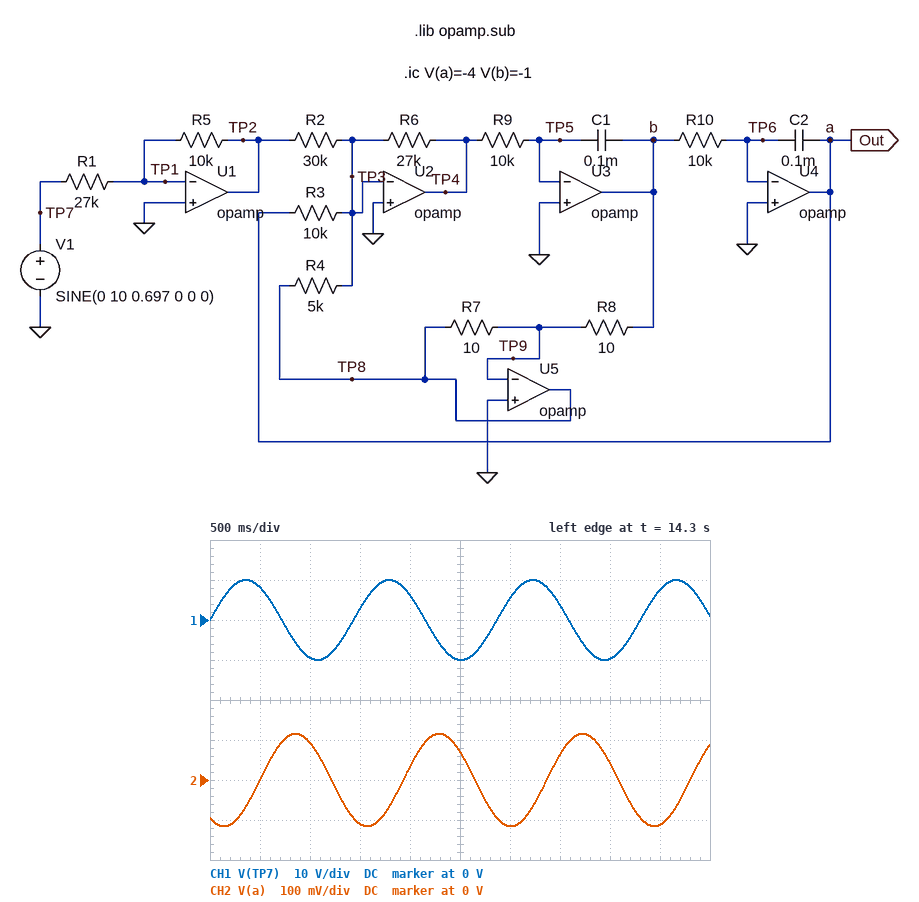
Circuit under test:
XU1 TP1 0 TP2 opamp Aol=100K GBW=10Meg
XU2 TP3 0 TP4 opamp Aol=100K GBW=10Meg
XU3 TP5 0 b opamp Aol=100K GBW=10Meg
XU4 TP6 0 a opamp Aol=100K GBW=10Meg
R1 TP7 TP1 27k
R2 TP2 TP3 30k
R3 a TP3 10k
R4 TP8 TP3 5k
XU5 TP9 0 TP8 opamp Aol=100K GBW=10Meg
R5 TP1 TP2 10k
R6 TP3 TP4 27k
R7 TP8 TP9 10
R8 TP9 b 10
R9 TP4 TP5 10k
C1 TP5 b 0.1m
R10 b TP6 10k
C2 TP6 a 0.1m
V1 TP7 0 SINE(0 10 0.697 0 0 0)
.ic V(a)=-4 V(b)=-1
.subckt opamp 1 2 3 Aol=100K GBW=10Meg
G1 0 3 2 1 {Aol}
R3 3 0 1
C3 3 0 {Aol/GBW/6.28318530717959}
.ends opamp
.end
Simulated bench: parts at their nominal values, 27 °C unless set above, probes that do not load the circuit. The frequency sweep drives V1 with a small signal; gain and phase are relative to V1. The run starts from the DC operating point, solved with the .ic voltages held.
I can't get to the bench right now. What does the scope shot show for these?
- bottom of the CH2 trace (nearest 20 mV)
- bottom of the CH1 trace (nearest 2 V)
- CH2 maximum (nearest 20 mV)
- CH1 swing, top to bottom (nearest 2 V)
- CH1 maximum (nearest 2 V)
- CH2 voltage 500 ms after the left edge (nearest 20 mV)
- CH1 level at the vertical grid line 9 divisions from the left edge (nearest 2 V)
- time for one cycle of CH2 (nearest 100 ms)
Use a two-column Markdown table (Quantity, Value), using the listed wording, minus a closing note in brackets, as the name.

| Quantity | Value |
|---|---|
| bottom of the CH2 trace | -120 mV |
| bottom of the CH1 trace | -10 V |
| CH2 maximum | 120 mV |
| CH1 swing, top to bottom | 20 V |
| CH1 maximum | 10 V |
| CH2 voltage 500 ms after the left edge | 0 V |
| CH1 level at the vertical grid line 9 divisions from the left edge | 8 V |
| time for one cycle of CH2 | 1.4 s |
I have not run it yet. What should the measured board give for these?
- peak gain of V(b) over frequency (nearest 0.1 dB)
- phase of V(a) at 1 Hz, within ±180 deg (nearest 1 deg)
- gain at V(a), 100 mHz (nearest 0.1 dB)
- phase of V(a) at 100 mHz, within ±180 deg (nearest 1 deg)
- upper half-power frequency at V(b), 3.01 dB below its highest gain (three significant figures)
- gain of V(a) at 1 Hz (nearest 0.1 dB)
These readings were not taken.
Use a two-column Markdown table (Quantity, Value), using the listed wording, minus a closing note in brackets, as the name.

| Quantity | Value |
|---|---|
| peak gain of V(b) over frequency | -24.2 dB |
| phase of V(a) at 1 Hz, within ±180 deg | -137 deg |
| gain at V(a), 100 mHz | -21.8 dB |
| phase of V(a) at 100 mHz, within ±180 deg | -56 deg |
| upper half-power frequency at V(b), 3.01 dB below its highest gain | 933 mHz |
| gain of V(a) at 1 Hz | -43.5 dB |
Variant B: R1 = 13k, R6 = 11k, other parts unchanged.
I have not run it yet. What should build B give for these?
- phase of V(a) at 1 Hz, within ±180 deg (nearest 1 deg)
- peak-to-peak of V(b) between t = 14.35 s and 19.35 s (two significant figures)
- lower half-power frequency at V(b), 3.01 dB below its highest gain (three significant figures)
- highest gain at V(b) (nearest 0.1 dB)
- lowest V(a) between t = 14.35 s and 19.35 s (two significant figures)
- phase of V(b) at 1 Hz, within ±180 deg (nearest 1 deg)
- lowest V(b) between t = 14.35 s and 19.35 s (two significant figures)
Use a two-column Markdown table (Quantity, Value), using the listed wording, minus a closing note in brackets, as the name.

| Quantity | Value |
|---|---|
| phase of V(a) at 1 Hz, within ±180 deg | -160 deg |
| peak-to-peak of V(b) between t = 14.35 s and 19.35 s | 1.2 V |
| lower half-power frequency at V(b), 3.01 dB below its highest gain | 66.8 mHz |
| highest gain at V(b) | -17.8 dB |
| lowest V(a) between t = 14.35 s and 19.35 s | -140 mV |
| phase of V(b) at 1 Hz, within ±180 deg | 110 deg |
| lowest V(b) between t = 14.35 s and 19.35 s | -600 mV |
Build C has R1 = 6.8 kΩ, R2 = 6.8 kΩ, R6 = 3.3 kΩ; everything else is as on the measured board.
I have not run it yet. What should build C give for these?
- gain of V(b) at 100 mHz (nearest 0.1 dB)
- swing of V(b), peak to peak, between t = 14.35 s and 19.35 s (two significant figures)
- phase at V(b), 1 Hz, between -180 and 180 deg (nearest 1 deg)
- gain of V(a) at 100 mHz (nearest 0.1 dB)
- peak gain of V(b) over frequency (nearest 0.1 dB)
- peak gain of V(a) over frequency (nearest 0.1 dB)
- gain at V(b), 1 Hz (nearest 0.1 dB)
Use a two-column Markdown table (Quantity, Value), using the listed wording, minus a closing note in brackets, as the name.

| Quantity | Value |
|---|---|
| gain of V(b) at 100 mHz | 0.6 dB |
| swing of V(b), peak to peak, between t = 14.35 s and 19.35 s | 3.3 V |
| phase at V(b), 1 Hz, between -180 and 180 deg | 96 deg |
| gain of V(a) at 100 mHz | 4.6 dB |
| peak gain of V(b) over frequency | 0.7 dB |
| peak gain of V(a) over frequency | 7.2 dB |
| gain at V(b), 1 Hz | -18.9 dB |
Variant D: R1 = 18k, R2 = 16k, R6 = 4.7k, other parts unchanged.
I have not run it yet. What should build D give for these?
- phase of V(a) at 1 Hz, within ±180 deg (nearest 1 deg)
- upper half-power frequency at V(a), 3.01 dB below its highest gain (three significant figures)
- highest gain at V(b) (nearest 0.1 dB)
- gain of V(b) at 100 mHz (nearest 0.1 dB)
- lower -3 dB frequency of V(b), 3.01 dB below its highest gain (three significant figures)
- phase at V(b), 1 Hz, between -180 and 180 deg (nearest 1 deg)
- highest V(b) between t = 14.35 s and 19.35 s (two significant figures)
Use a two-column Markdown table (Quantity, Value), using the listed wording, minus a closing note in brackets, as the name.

| Quantity | Value |
|---|---|
| phase of V(a) at 1 Hz, within ±180 deg | -171 deg |
| upper half-power frequency at V(a), 3.01 dB below its highest gain | 112 mHz |
| highest gain at V(b) | -15.2 dB |
| gain of V(b) at 100 mHz | -15.3 dB |
| lower -3 dB frequency of V(b), 3.01 dB below its highest gain | 57.5 mHz |
| phase at V(b), 1 Hz, between -180 and 180 deg | 99 deg |
| highest V(b) between t = 14.35 s and 19.35 s | 370 mV |
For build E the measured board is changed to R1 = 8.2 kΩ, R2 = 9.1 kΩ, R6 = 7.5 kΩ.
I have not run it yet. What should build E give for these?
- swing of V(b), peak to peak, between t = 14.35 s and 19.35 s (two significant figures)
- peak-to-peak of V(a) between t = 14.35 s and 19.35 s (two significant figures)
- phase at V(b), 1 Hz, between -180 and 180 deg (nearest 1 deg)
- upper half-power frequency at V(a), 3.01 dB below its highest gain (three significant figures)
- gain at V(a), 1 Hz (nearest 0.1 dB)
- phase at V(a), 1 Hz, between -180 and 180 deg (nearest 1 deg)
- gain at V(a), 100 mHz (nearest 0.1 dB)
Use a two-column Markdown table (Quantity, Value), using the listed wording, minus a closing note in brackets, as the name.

| Quantity | Value |
|---|---|
| swing of V(b), peak to peak, between t = 14.35 s and 19.35 s | 4.5 V |
| peak-to-peak of V(a) between t = 14.35 s and 19.35 s | 1.0 V |
| phase at V(b), 1 Hz, between -180 and 180 deg | 104 deg |
| upper half-power frequency at V(a), 3.01 dB below its highest gain | 108 mHz |
| gain at V(a), 1 Hz | -32.0 dB |
| phase at V(a), 1 Hz, between -180 and 180 deg | -166 deg |
| gain at V(a), 100 mHz | 0 dB |
